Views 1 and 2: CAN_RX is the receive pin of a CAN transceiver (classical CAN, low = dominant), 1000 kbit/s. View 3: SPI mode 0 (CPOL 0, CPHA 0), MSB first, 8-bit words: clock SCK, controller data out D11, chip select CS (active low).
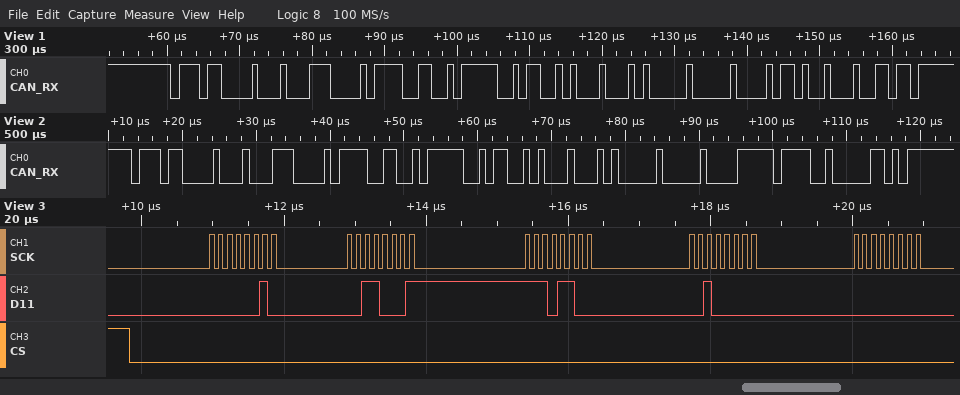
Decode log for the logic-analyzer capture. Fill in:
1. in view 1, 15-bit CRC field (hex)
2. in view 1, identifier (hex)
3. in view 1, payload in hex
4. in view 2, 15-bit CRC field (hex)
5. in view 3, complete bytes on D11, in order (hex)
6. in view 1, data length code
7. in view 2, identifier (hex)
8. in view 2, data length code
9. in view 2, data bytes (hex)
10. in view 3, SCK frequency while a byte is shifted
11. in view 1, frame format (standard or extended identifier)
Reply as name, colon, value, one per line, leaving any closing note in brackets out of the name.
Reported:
in view 1, 15-bit CRC field: 0x244D
in view 1, identifier: 0x761
in view 1, payload in hex: E1 79 97 D6 51 14 00 0B
in view 2, 15-bit CRC field: 0x7C82
in view 3, complete bytes on D11, in order: 02 31 EC 20 00
in view 1, data length code: 8
in view 2, identifier: 0x761
in view 2, data length code: 8
in view 2, data bytes: E1 79 97 D6 51 14 00 0F
in view 3, SCK frequency while a byte is shifted: 8 MHz
in view 1, frame format: standard
